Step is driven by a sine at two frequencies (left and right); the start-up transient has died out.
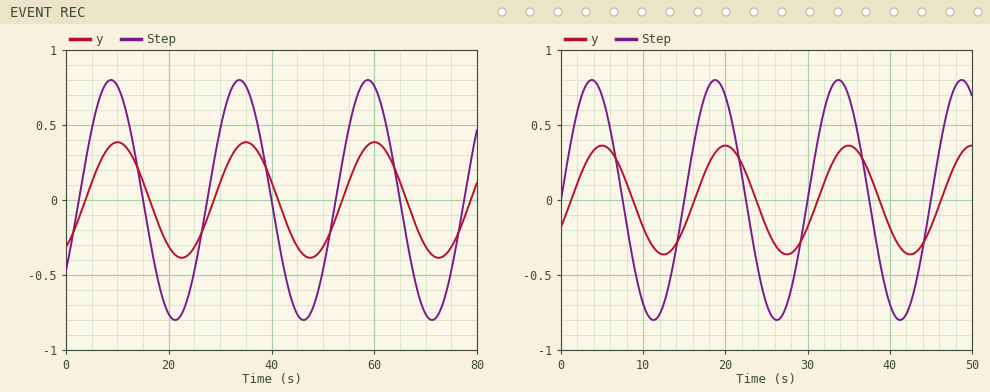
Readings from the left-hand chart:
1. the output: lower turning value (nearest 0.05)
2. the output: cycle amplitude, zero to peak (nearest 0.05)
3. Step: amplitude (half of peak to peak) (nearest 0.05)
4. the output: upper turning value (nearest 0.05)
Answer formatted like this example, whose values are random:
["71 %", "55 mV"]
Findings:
["-0.40", "0.40", "0.80", "0.40"]
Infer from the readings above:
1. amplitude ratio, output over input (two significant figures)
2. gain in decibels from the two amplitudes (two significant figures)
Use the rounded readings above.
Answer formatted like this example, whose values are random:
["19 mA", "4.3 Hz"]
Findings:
["0.50", "-6.0 dB"]
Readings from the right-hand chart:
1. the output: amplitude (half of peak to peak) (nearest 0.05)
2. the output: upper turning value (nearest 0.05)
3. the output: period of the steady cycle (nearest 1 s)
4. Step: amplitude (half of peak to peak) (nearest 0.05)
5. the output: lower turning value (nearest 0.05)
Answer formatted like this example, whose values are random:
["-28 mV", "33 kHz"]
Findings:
["0.35", "0.35", "15 s", "0.80", "-0.35"]
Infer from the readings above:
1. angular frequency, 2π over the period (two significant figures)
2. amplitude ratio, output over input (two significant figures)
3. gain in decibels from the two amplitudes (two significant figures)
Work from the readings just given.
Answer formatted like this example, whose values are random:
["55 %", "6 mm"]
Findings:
["0.42 rad/s", "0.44", "-7.2 dB"]
